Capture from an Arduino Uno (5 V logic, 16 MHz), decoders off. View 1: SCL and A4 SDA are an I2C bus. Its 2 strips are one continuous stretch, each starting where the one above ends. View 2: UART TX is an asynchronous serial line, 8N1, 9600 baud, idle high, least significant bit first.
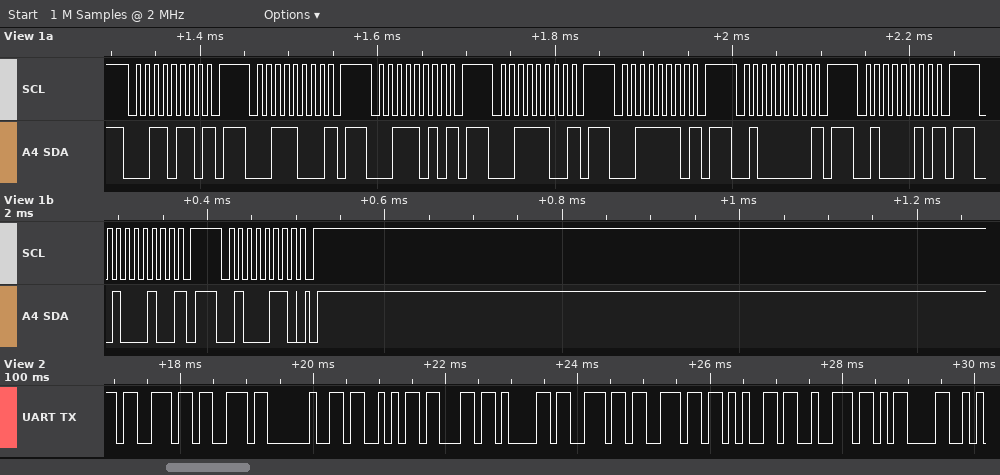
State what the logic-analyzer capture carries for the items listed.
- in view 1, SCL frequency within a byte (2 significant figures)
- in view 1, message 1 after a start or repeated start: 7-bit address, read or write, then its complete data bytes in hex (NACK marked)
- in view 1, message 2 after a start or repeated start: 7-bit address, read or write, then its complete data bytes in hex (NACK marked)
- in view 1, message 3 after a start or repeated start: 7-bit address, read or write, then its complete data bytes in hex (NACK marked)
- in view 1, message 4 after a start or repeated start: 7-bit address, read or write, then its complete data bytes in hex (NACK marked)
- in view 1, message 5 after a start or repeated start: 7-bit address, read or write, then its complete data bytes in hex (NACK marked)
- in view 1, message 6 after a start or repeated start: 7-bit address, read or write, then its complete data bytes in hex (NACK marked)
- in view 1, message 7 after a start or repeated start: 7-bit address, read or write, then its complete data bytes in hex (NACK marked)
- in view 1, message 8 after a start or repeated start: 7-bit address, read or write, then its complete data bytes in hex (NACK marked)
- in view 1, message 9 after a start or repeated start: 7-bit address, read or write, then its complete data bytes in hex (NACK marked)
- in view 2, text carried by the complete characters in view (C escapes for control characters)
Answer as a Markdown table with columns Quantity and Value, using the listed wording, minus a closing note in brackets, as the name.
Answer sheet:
| Quantity | Value |
|---|---|
| in view 1, SCL frequency within a byte | 100 kHz |
| in view 1, message 1 after a start or repeated start: 7-bit address, read or write, then its complete data bytes in hex | 0x1B write NACK |
| in view 1, message 2 after a start or repeated start: 7-bit address, read or write, then its complete data bytes in hex | 0x1C write NACK |
| in view 1, message 3 after a start or repeated start: 7-bit address, read or write, then its complete data bytes in hex | 0x1D write NACK |
| in view 1, message 4 after a start or repeated start: 7-bit address, read or write, then its complete data bytes in hex | 0x1E write NACK |
| in view 1, message 5 after a start or repeated start: 7-bit address, read or write, then its complete data bytes in hex | 0x1F write NACK |
| in view 1, message 6 after a start or repeated start: 7-bit address, read or write, then its complete data bytes in hex | 0x20 write NACK |
| in view 1, message 7 after a start or repeated start: 7-bit address, read or write, then its complete data bytes in hex | 0x21 write NACK |
| in view 1, message 8 after a start or repeated start: 7-bit address, read or write, then its complete data bytes in hex | 0x22 write NACK |
| in view 1, message 9 after a start or repeated start: 7-bit address, read or write, then its complete data bytes in hex | 0x23 write |
| in view 2, text carried by the complete characters in view | "ss Scanner\r" |
